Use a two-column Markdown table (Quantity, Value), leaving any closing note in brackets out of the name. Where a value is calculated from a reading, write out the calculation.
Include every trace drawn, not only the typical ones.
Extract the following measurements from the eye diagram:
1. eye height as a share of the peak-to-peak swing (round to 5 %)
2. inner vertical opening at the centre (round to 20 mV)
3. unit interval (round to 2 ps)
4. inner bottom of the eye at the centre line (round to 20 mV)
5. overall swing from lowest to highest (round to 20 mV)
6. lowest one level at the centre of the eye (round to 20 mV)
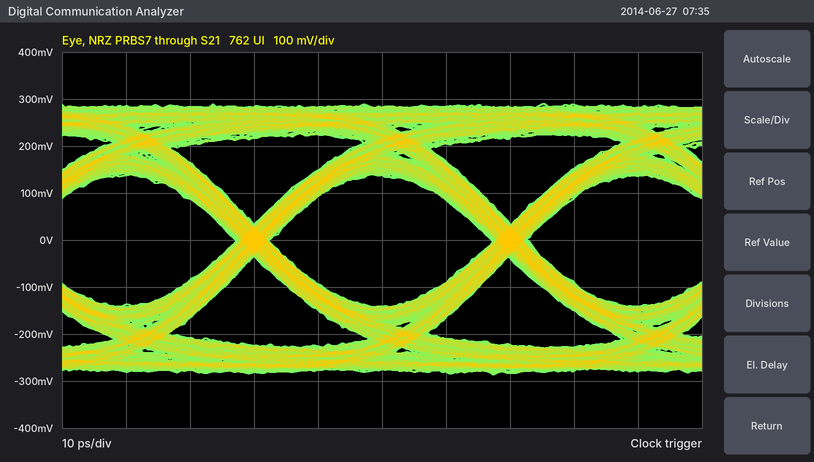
| Quantity | Value |
|---|---|
| eye height as a share of the peak-to-peak swing | 280 mV / 580 mV ≈ 48.3 %, so 50 % to the nearest 5 % |
| inner vertical opening at the centre | 280 mV |
| unit interval | 40 ps |
| inner bottom of the eye at the centre line | -140 mV |
| overall swing from lowest to highest | 580 mV |
| lowest one level at the centre of the eye | 140 mV |
